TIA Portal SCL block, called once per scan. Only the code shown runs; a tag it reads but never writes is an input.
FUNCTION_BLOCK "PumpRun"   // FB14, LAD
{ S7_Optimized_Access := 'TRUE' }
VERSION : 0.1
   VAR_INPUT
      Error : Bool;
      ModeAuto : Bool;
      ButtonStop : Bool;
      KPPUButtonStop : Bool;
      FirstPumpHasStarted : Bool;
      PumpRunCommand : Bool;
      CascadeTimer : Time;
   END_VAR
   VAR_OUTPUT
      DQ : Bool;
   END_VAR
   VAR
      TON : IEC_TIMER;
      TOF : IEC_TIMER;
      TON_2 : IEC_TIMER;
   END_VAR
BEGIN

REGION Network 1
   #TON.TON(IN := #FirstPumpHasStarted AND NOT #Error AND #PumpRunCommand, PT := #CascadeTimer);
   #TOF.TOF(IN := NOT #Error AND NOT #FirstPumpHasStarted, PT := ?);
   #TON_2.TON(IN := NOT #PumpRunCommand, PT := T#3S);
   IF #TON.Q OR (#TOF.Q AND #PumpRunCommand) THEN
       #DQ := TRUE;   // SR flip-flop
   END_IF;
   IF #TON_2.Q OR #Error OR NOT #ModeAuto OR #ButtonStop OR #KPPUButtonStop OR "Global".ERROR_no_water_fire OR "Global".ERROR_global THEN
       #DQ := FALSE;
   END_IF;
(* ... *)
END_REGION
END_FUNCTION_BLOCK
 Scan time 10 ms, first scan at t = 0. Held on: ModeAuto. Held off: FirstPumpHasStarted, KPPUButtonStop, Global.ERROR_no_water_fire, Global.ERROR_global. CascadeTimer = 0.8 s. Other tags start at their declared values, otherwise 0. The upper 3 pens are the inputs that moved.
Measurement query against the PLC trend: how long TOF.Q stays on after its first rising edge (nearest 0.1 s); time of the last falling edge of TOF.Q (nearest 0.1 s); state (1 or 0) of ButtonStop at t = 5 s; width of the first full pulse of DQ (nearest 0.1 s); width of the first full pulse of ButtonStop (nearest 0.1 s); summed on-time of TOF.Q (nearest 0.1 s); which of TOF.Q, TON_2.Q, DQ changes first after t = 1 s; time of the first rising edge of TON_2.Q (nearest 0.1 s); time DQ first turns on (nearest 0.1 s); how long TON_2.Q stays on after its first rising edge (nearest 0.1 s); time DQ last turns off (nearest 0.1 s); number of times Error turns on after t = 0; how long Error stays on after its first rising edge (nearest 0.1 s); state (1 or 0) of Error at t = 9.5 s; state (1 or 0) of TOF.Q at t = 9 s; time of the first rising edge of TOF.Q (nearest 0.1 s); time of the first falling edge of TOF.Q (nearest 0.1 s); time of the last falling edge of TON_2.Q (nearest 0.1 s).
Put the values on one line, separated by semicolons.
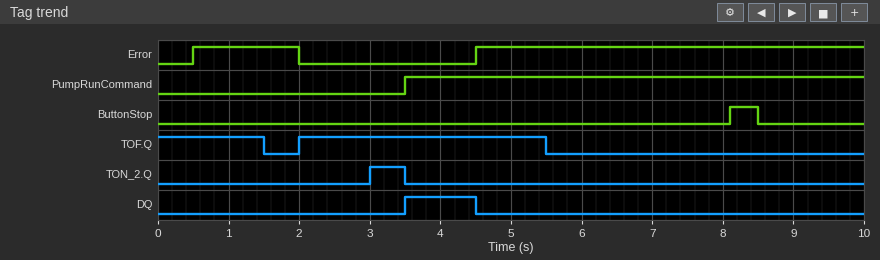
3.5 s; 5.5 s; 0; 1.0 s; 0.4 s; 5.0 s; TOF.Q; 3.0 s; 3.5 s; 0.5 s; 4.5 s; 2; 1.5 s; 1; 0; 2.0 s; 1.5 s; 3.5 s
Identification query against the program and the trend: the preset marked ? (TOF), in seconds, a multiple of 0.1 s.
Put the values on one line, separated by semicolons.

1.0 s
